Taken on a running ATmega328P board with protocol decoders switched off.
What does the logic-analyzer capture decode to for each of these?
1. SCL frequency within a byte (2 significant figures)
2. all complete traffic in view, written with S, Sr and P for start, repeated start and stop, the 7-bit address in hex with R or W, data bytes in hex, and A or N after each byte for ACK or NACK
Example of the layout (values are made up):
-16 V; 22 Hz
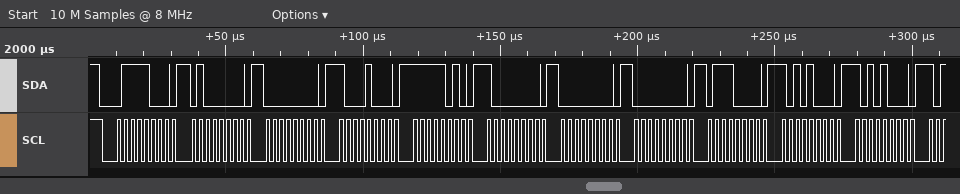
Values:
400 kHz; S 3CW A 40 A 00 A 88 A FA A 80 A 00 A 00 A 70 A A8 A A8 A
